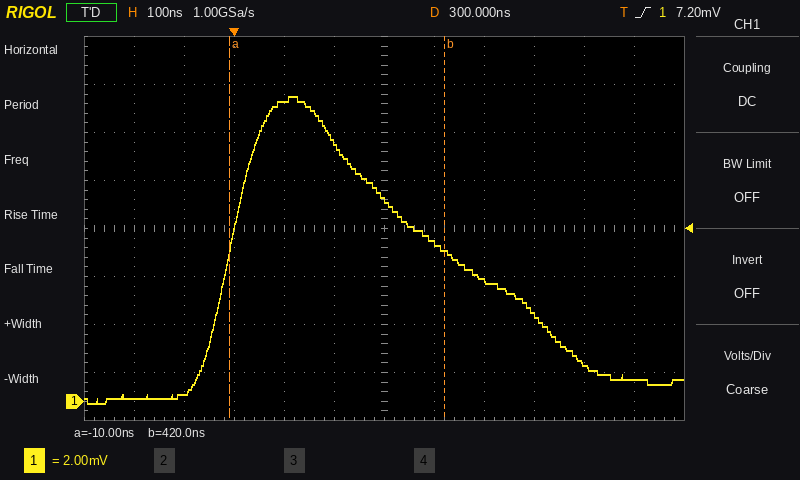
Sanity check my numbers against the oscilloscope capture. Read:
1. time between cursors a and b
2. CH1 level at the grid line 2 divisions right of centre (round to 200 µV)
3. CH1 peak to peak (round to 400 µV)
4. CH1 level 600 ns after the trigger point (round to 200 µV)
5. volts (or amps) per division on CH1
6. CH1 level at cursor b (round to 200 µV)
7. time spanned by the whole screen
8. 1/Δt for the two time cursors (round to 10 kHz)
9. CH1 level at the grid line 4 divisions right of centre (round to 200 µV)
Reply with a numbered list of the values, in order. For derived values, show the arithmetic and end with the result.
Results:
1. 420 ns − (-10 ns) = 430 ns
2. 5.0 mV
3. 12.8 mV
4. 3.6 mV
5. 2 mV
6. 6.2 mV
7. 1.2 µs
8. 1 / 430 ns ≈ 2.33 MHz
9. 1.6 mV
